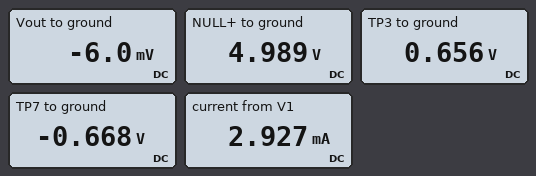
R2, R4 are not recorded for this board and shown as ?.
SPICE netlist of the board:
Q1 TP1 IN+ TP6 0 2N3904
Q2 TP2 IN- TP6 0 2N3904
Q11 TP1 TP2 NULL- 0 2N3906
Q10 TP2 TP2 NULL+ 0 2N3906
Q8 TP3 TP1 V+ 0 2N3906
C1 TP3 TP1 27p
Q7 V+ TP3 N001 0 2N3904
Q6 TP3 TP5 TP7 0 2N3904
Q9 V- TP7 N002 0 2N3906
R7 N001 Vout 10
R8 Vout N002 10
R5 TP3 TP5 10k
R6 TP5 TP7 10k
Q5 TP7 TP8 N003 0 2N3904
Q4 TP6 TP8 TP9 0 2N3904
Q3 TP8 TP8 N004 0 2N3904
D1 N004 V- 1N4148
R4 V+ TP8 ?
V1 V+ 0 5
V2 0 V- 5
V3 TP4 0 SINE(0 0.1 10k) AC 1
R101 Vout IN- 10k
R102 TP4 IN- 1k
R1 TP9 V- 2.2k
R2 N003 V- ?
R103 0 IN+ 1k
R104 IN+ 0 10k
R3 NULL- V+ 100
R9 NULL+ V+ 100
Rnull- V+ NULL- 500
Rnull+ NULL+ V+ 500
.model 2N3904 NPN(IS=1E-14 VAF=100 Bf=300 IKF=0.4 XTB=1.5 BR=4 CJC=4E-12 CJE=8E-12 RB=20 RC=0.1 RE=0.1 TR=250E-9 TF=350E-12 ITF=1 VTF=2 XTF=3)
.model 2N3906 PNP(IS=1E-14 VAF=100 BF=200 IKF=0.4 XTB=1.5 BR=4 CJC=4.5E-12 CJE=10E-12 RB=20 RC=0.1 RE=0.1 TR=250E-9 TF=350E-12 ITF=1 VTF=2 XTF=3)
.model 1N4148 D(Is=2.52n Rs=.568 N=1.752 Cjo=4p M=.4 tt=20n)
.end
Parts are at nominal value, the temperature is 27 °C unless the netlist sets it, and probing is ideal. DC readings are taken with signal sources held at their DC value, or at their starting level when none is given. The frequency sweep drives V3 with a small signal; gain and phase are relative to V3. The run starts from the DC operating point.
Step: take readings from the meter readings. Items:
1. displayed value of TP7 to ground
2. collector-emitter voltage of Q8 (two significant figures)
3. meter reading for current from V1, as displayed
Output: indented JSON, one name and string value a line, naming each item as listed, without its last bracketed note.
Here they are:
{
  "displayed value of TP7 to ground": "-0.668 V",
  "collector-emitter voltage of Q8": "-4.3 V",
  "meter reading for current from V1, as displayed": "2.927 mA"
}
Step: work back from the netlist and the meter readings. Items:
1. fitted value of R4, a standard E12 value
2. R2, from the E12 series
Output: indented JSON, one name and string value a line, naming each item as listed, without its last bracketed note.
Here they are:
{
  "fitted value of R4, a standard E12 value": "10 kΩ",
  "R2, from the E12 series": "680 Ω"
}
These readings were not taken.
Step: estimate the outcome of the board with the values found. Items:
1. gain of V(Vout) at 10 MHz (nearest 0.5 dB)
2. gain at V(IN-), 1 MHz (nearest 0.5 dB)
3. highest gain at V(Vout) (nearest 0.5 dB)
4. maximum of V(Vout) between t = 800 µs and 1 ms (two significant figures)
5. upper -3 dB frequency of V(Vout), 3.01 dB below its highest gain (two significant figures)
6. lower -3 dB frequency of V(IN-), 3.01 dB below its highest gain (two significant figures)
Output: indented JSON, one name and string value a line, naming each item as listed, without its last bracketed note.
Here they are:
{
  "gain of V(Vout) at 10 MHz": "5.5 dB",
  "gain at V(IN-), 1 MHz": "-9.0 dB",
  "highest gain at V(Vout)": "20.0 dB",
  "maximum of V(Vout) between t = 800 µs and 1 ms": "990 mV",
  "upper -3 dB frequency of V(Vout), 3.01 dB below its highest gain": "3.9 MHz",
  "lower -3 dB frequency of V(IN-), 3.01 dB below its highest gain": "2.3 MHz"
}
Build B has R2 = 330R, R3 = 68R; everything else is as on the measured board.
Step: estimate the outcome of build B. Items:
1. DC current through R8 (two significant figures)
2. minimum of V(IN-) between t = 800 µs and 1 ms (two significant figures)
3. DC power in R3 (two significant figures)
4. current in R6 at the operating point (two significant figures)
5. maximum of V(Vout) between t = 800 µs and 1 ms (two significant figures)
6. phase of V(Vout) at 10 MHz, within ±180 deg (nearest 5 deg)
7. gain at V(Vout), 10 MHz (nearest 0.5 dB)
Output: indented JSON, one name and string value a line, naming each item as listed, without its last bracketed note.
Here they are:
{
  "DC current through R8": "2.1 mA",
  "minimum of V(IN-) between t = 800 µs and 1 ms": "-4.3 mV",
  "DC power in R3": "1.0 µW",
  "current in R6 at the operating point": "67 µA",
  "maximum of V(Vout) between t = 800 µs and 1 ms": "960 mV",
  "phase of V(Vout) at 10 MHz, within ±180 deg": "25 deg",
  "gain at V(Vout), 10 MHz": "6.0 dB"
}
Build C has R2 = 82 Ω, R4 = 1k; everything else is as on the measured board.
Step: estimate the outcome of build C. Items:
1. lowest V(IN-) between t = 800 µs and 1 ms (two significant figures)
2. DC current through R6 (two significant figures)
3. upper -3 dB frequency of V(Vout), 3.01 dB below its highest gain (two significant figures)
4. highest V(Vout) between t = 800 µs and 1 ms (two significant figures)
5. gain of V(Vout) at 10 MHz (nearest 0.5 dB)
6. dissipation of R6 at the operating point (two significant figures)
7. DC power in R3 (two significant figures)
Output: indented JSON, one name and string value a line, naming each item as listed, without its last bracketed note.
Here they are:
{
  "lowest V(IN-) between t = 800 µs and 1 ms": "-6.8 mV",
  "DC current through R6": "71 µA",
  "upper -3 dB frequency of V(Vout), 3.01 dB below its highest gain": "4.8 MHz",
  "highest V(Vout) between t = 800 µs and 1 ms": "930 mV",
  "gain of V(Vout) at 10 MHz": "7.5 dB",
  "dissipation of R6 at the operating point": "51 µW",
  "DC power in R3": "1.6 µW"
}
